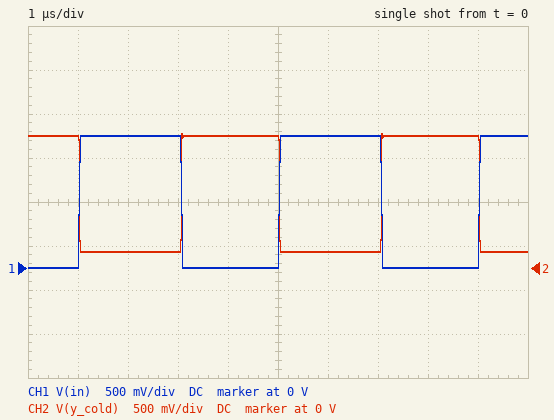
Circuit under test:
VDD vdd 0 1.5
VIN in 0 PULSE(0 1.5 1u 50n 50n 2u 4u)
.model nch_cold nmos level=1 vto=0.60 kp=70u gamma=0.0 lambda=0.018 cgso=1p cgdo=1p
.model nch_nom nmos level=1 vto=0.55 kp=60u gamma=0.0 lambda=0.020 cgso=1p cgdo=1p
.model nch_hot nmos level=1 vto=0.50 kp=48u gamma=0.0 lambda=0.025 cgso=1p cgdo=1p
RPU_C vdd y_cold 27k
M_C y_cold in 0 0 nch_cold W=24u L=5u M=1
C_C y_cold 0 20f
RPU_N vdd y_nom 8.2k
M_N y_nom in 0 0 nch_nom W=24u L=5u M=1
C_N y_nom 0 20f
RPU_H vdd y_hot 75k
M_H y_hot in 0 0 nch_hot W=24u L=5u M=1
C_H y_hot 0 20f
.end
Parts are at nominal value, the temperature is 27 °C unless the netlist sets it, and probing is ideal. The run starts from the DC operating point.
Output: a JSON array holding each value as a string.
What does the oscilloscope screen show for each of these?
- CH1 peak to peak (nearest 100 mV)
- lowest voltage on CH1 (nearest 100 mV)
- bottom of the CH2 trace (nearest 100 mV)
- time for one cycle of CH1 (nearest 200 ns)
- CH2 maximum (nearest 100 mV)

["1.5 V", "0 V", "200 mV", "4.0 µs", "1.5 V"]
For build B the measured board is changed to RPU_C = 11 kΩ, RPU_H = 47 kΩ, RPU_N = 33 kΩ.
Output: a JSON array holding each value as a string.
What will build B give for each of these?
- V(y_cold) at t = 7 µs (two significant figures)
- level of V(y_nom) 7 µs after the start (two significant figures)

["420 mV", "160 mV"]
